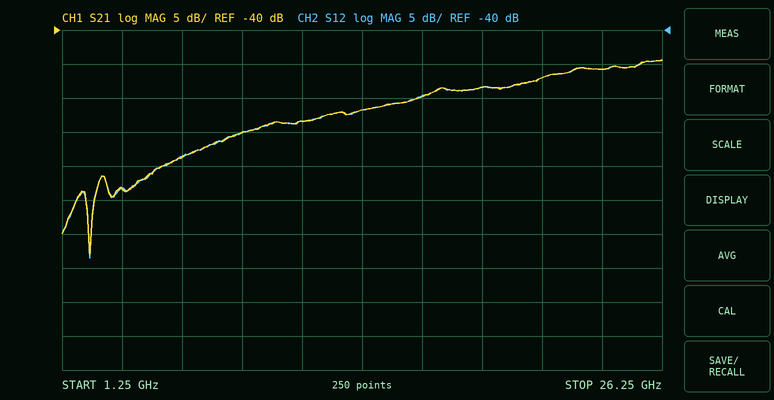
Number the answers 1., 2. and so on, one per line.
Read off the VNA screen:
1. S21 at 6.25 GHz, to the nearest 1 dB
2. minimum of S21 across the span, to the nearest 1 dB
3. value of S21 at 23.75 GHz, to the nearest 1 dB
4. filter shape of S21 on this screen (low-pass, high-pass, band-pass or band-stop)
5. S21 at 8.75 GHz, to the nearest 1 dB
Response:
1. -59 dB
2. -73 dB
3. -46 dB
4. high-pass
5. -55 dB
